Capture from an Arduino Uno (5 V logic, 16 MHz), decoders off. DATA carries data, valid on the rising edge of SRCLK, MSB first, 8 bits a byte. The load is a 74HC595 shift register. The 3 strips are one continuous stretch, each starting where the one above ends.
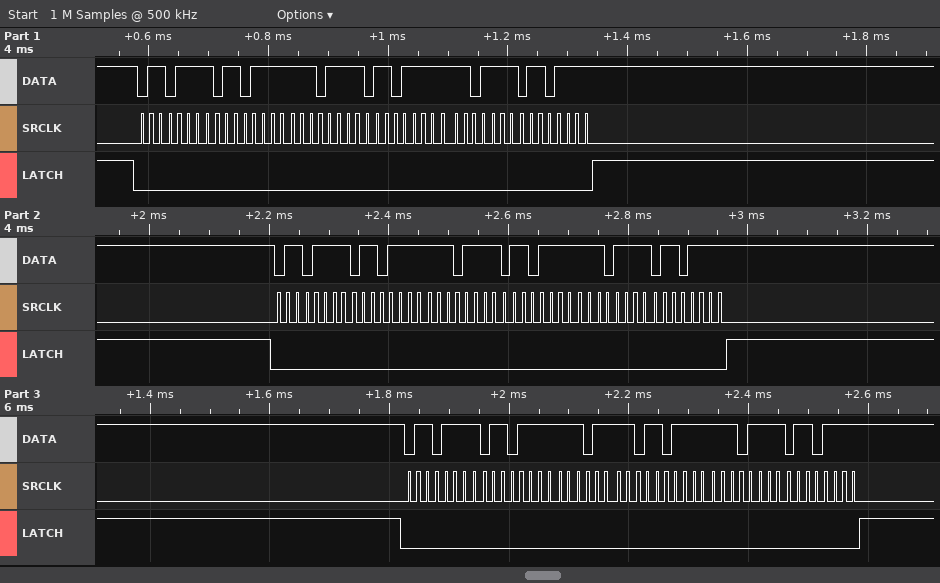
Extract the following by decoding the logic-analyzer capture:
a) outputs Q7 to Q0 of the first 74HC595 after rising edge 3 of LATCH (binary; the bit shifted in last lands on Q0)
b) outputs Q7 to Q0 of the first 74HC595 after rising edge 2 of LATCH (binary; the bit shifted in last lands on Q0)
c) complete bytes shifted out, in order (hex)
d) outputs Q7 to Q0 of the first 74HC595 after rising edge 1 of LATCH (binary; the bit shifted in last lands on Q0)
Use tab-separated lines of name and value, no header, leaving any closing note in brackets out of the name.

outputs Q7 to Q0 of the first 74HC595 after rising edge 3 of LATCH	01101111
outputs Q7 to Q0 of the first 74HC595 after rising edge 2 of LATCH	01101111
complete bytes shifted out, in order	6F 6F EF 6F EF 6F 6F 6F EF 6F EF 6F 6F 6F EF 6F EF 6F
outputs Q7 to Q0 of the first 74HC595 after rising edge 1 of LATCH	01101111
